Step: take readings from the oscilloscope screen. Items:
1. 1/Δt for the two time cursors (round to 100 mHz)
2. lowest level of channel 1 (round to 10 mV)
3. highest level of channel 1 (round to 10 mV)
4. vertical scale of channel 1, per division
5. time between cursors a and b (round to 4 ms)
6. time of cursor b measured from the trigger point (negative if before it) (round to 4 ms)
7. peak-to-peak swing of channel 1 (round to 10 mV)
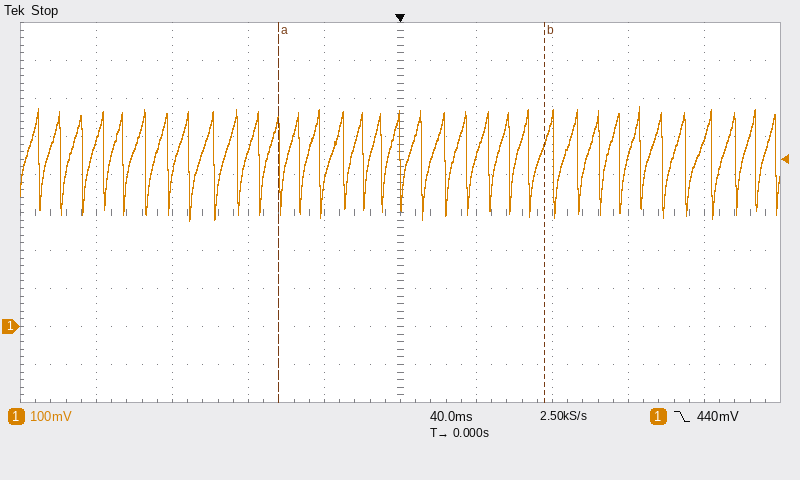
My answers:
7.1 Hz
280 mV
580 mV
100 mV
140 ms
+76 ms
300 mV
